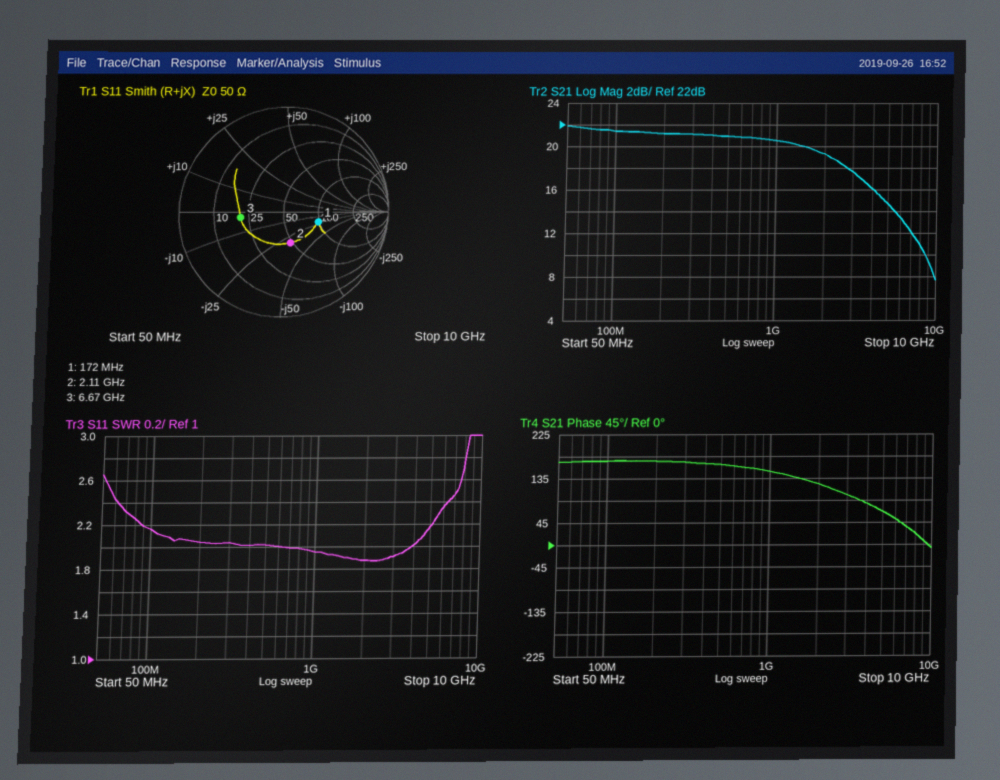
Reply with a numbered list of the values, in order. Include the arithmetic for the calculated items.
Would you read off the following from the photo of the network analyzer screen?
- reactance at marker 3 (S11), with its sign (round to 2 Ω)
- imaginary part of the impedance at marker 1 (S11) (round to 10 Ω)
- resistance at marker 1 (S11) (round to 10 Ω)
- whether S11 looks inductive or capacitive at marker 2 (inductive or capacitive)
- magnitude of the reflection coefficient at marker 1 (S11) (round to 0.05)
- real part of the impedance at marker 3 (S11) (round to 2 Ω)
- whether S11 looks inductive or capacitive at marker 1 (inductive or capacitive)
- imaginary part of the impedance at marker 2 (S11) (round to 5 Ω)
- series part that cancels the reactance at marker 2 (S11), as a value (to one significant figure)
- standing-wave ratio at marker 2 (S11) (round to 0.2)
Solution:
1. -2 Ω
2. -20 Ω
3. 100 Ω
4. capacitive
5. 0.35
6. 20 Ω
7. capacitive
8. -30 Ω
9. L = 30 Ω/(2π × 2.11 GHz) ≈ 2 nH
10. 1.8
